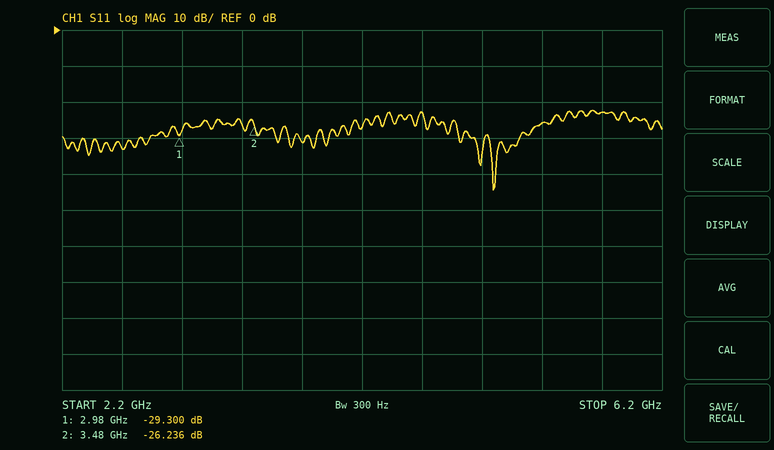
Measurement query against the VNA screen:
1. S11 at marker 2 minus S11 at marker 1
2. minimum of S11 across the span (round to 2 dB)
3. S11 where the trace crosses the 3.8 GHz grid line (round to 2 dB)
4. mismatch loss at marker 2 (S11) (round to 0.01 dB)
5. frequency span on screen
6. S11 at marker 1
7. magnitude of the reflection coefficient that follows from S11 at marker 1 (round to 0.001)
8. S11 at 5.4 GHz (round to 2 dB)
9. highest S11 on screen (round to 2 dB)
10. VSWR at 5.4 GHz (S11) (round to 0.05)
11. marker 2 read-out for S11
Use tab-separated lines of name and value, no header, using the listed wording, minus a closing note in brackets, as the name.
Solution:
S11 at marker 2 minus S11 at marker 1	3.064 dB
minimum of S11 across the span	-44 dB
S11 where the trace crosses the 3.8 GHz grid line	-32 dB
mismatch loss at marker 2 (S11)	0.01 dB
frequency span on screen	4 GHz
S11 at marker 1	-29.300 dB
magnitude of the reflection coefficient that follows from S11 at marker 1	0.034
S11 at 5.4 GHz	-26 dB
highest S11 on screen	-22 dB
VSWR at 5.4 GHz (S11)	1.10
marker 2 read-out for S11	-26.236 dB
